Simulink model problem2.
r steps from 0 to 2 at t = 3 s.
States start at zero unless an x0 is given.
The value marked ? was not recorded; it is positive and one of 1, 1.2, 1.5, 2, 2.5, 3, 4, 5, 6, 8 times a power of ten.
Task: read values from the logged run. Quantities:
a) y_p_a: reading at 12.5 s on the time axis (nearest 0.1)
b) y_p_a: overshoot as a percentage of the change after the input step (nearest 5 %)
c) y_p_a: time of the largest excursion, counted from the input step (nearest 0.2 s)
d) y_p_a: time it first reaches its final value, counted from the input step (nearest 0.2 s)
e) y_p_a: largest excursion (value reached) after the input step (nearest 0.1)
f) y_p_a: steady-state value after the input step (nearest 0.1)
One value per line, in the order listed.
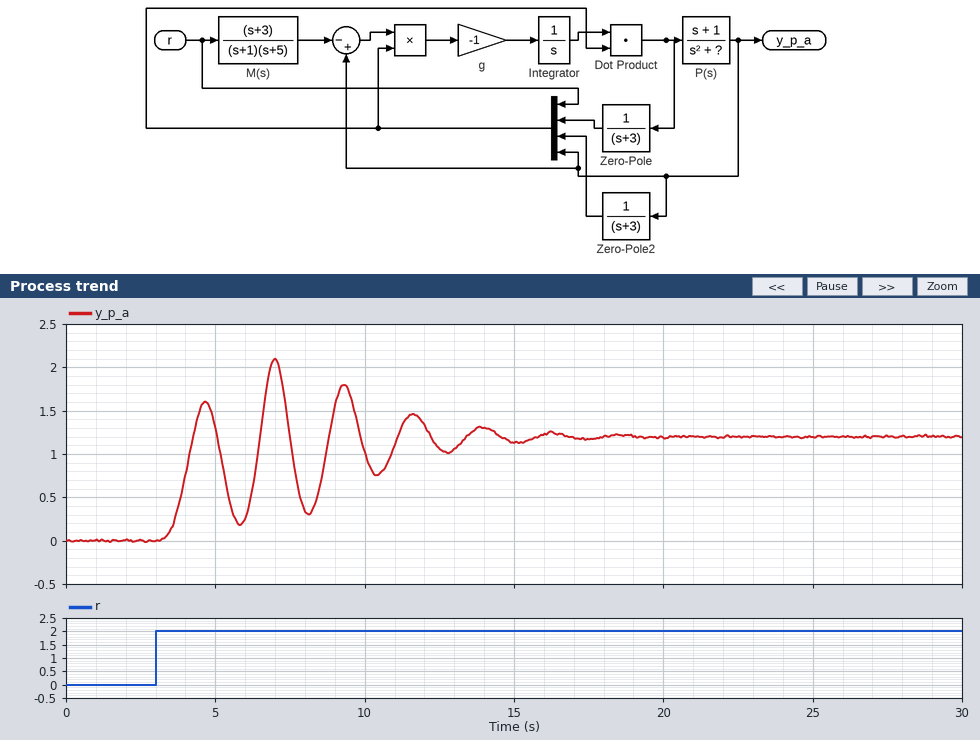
1.1
75 %
4.0 s
1.2 s
2.1
1.2
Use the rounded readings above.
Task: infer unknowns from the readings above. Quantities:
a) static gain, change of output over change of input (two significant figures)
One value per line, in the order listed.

0.60
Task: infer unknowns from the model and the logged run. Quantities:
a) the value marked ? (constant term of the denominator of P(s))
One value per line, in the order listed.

1
